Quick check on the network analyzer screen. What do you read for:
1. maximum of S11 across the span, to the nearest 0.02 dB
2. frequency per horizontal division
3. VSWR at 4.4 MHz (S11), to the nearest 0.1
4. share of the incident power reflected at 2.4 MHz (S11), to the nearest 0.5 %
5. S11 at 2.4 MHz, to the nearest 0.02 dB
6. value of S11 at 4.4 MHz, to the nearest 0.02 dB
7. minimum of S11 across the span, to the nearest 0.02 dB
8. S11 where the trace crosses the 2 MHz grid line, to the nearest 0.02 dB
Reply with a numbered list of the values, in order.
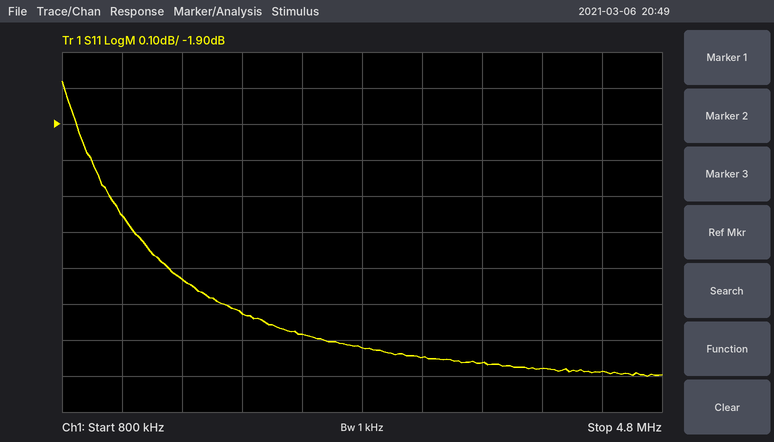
1. -1.78 dB
2. 400 kHz
3. 6.8
4. 56.5 %
5. -2.48 dB
6. -2.58 dB
7. -2.60 dB
8. -2.42 dB
